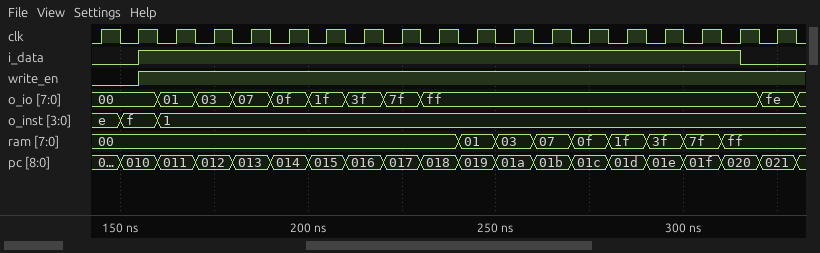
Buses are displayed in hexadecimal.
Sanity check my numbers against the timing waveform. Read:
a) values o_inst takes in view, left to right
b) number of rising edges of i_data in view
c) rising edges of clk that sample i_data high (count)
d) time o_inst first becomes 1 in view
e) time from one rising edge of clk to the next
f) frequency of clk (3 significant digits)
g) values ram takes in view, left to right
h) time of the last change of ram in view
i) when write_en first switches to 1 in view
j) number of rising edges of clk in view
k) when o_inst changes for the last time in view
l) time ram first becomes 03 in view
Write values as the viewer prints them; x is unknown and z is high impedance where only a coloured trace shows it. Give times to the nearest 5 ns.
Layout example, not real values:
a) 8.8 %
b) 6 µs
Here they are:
a) e, f, 1
b) 1
c) 16
d) 160 ns
e) 10 ns
f) 100 MHz
g) 00, 01, 03, 07, 0f, 1f, 3f, 7f, ff
h) 310 ns
i) 155 ns
j) 19
k) 160 ns
l) 250 ns
